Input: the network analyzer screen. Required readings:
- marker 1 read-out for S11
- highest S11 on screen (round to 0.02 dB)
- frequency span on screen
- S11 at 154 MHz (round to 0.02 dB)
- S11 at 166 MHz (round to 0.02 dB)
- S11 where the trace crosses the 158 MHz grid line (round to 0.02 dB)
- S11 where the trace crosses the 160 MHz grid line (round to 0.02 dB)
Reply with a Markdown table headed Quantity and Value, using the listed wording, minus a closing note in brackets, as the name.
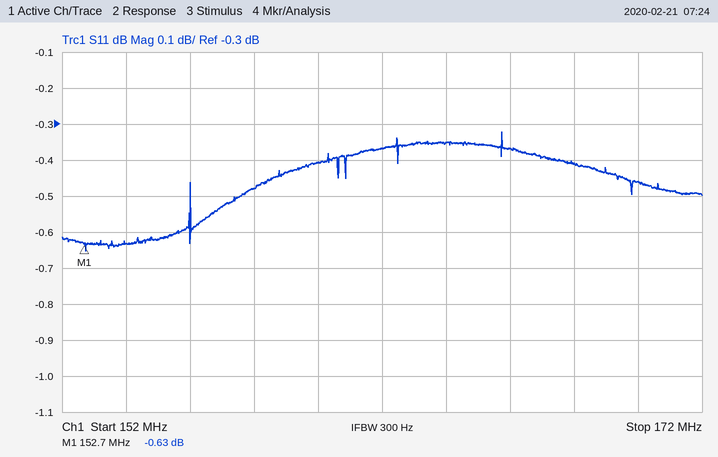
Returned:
| Quantity | Value |
|---|---|
| marker 1 read-out for S11 | -0.63 dB |
| highest S11 on screen | -0.32 dB |
| frequency span on screen | 20 MHz |
| S11 at 154 MHz | -0.64 dB |
| S11 at 166 MHz | -0.36 dB |
| S11 where the trace crosses the 158 MHz grid line | -0.48 dB |
| S11 where the trace crosses the 160 MHz grid line | -0.40 dB |
